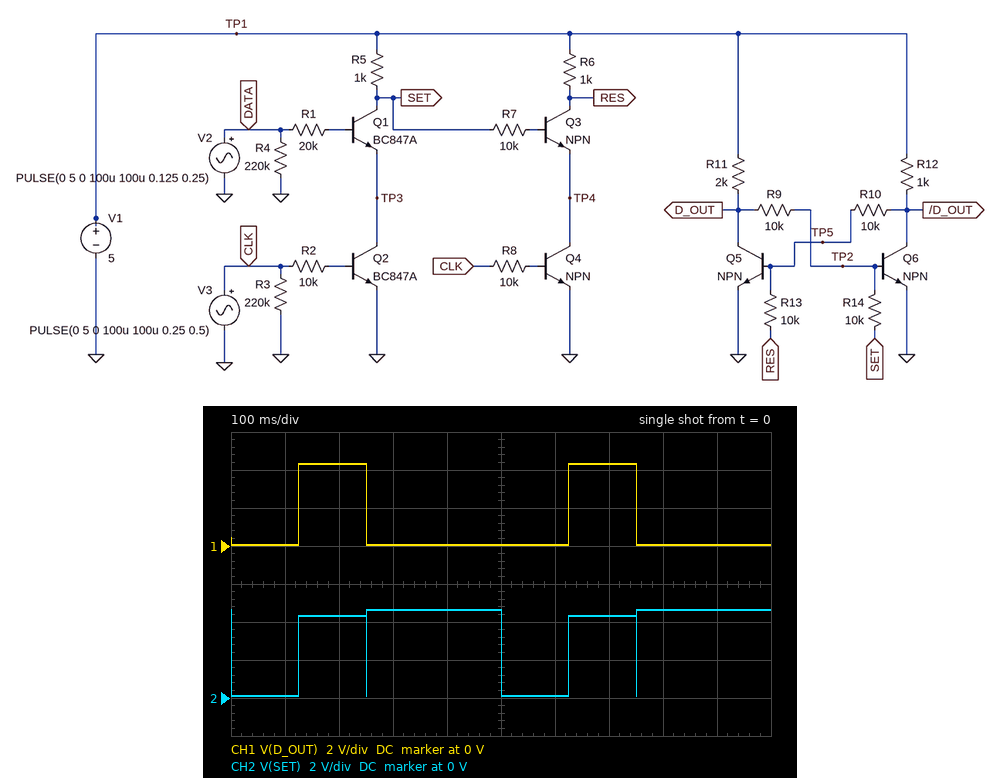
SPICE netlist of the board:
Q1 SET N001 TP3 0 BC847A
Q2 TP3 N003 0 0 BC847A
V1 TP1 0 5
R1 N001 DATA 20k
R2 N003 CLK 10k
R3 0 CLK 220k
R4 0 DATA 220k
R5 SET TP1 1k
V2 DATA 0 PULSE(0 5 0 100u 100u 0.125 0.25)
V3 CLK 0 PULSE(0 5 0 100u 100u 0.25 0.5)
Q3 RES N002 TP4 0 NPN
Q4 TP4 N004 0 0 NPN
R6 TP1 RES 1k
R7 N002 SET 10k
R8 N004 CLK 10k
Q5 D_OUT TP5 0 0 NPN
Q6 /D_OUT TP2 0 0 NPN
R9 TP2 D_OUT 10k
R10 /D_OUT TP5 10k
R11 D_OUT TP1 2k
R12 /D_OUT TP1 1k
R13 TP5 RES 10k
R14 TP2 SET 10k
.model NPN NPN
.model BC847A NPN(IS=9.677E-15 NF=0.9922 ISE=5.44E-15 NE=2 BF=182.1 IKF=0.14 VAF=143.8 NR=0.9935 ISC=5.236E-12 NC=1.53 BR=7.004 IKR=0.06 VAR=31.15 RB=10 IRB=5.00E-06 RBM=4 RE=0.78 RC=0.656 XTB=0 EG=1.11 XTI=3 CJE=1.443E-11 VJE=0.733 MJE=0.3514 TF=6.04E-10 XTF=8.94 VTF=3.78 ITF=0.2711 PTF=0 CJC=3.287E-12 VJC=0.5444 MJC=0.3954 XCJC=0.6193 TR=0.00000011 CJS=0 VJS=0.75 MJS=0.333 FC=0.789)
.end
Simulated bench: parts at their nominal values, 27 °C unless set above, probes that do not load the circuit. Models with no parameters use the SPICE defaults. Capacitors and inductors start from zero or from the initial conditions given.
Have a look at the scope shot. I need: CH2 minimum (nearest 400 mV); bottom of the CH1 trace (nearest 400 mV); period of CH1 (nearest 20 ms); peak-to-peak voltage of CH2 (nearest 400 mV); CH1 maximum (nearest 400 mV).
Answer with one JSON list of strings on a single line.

["0 V", "0 V", "500 ms", "4.4 V", "4.4 V"]
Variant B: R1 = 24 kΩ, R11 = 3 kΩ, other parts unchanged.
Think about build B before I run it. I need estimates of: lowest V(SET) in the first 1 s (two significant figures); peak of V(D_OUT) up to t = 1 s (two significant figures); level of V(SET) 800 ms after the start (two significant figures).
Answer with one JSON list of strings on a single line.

["110 mV", "4.0 V", "4.6 V"]
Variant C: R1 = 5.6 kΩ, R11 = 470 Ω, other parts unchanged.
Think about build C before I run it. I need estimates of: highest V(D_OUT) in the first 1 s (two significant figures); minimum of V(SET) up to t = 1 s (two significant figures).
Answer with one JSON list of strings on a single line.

["4.8 V", "79 mV"]
